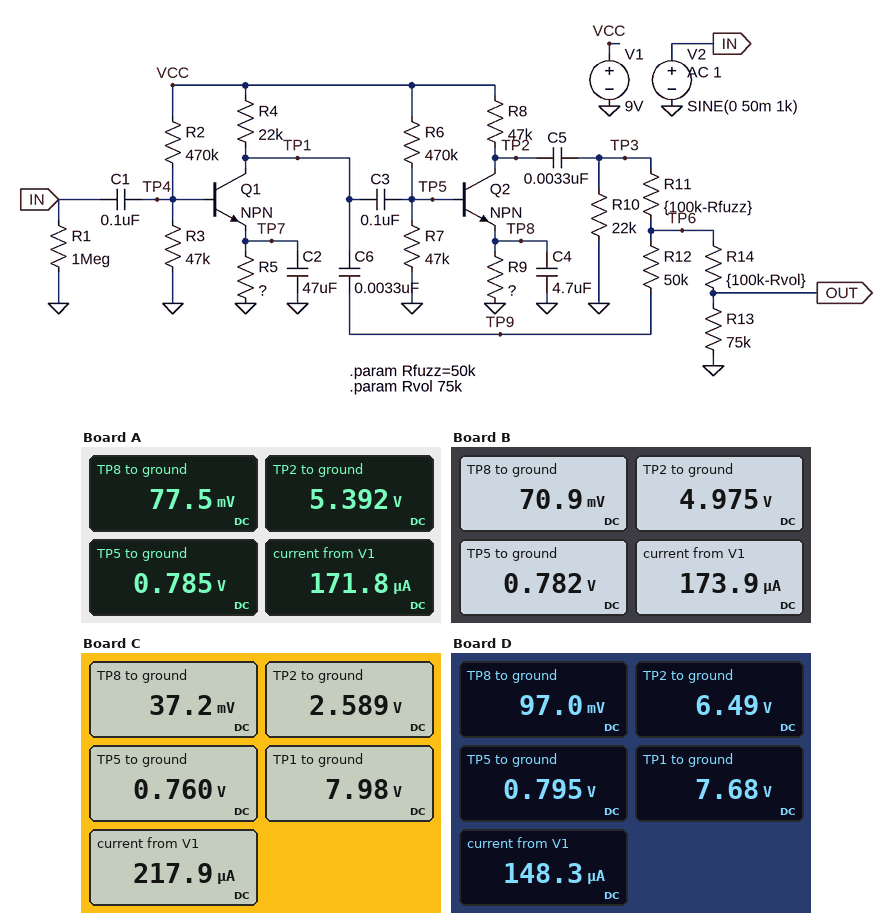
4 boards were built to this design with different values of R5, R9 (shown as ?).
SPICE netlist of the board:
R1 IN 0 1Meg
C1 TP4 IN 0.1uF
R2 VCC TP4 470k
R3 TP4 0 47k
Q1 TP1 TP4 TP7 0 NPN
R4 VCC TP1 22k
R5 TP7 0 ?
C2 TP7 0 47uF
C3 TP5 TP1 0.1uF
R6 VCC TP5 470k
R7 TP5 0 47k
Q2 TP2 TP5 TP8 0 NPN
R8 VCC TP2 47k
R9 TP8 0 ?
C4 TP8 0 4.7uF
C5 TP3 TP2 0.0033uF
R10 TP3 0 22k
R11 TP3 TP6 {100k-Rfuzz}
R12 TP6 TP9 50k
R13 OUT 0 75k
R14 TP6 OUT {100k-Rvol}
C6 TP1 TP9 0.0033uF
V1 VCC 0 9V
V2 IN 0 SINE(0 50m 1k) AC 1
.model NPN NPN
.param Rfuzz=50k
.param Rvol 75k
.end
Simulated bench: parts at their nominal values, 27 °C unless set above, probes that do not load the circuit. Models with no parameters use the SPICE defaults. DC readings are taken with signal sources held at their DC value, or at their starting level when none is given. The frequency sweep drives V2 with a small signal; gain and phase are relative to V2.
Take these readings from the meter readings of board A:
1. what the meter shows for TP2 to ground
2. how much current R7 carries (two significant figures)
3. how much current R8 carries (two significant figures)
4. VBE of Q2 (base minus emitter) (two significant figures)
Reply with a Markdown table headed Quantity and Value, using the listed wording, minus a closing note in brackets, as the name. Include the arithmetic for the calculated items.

| Quantity | Value |
|---|---|
| what the meter shows for TP2 to ground | 5.392 V |
| how much current R7 carries | (785 mV) / 47 kΩ = 17 µA |
| how much current R8 carries | (9 V - 5.392 V) / 47 kΩ = 77 µA |
| VBE of Q2 (base minus emitter) | 785 mV - 77.5 mV = 710 mV |
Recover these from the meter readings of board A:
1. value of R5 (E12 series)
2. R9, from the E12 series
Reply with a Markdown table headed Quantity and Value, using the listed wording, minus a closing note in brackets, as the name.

| Quantity | Value |
|---|---|
| value of R5 | 1.5 kΩ |
| R9, from the E12 series | 1 kΩ |
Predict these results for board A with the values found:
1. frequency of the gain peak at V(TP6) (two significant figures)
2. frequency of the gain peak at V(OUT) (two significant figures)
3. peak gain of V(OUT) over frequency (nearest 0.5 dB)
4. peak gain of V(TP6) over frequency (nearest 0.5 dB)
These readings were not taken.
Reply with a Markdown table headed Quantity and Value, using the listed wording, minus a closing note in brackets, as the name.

| Quantity | Value |
|---|---|
| frequency of the gain peak at V(TP6) | 340 Hz |
| frequency of the gain peak at V(OUT) | 340 Hz |
| peak gain of V(OUT) over frequency | 47.0 dB |
| peak gain of V(TP6) over frequency | 49.5 dB |
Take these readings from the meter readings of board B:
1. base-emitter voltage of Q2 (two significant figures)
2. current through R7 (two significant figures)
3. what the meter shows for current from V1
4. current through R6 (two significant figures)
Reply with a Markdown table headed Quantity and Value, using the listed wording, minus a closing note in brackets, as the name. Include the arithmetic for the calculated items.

| Quantity | Value |
|---|---|
| base-emitter voltage of Q2 | 782 mV - 70.9 mV = 710 mV |
| current through R7 | (782 mV) / 47 kΩ = 17 µA |
| what the meter shows for current from V1 | 173.9 µA |
| current through R6 | (9 V - 782 mV) / 470 kΩ = 17 µA |
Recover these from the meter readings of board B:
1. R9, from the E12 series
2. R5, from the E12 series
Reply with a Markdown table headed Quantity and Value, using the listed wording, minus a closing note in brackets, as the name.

| Quantity | Value |
|---|---|
| R9, from the E12 series | 820 Ω |
| R5, from the E12 series | 1.8 kΩ |
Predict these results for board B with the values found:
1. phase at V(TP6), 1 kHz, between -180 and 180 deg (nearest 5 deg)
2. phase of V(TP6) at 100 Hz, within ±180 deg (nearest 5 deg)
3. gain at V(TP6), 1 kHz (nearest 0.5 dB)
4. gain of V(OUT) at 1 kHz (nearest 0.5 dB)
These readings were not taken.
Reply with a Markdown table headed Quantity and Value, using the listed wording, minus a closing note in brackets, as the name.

| Quantity | Value |
|---|---|
| phase at V(TP6), 1 kHz, between -180 and 180 deg | -20 deg |
| phase of V(TP6) at 100 Hz, within ±180 deg | 165 deg |
| gain at V(TP6), 1 kHz | 41.0 dB |
| gain of V(OUT) at 1 kHz | 38.5 dB |
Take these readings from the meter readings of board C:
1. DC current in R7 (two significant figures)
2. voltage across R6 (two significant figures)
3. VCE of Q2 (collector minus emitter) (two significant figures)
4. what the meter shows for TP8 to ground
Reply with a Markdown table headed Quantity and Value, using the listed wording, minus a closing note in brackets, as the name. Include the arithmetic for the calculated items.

| Quantity | Value |
|---|---|
| DC current in R7 | (760 mV) / 47 kΩ = 16 µA |
| voltage across R6 | 9 V - 760 mV = 8.2 V |
| VCE of Q2 (collector minus emitter) | 2.589 V - 37.2 mV = 2.6 V |
| what the meter shows for TP8 to ground | 37.2 mV |
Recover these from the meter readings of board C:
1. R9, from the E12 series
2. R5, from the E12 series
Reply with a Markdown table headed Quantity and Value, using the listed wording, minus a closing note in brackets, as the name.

| Quantity | Value |
|---|---|
| R9, from the E12 series | 270 Ω |
| R5, from the E12 series | 2.2 kΩ |
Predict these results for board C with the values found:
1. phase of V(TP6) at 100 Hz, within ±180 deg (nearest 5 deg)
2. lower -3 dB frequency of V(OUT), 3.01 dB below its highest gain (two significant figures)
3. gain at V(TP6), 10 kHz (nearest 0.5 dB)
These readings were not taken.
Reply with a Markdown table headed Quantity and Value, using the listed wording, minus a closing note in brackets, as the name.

| Quantity | Value |
|---|---|
| phase of V(TP6) at 100 Hz, within ±180 deg | 150 deg |
| lower -3 dB frequency of V(OUT), 3.01 dB below its highest gain | 240 Hz |
| gain at V(TP6), 10 kHz | 37.0 dB |
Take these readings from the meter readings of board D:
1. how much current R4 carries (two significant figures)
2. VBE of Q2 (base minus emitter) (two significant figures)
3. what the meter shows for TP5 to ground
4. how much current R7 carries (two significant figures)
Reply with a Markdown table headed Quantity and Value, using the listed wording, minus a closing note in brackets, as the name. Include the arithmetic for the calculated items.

| Quantity | Value |
|---|---|
| how much current R4 carries | (9 V - 7.68 V) / 22 kΩ = 60 µA |
| VBE of Q2 (base minus emitter) | 795 mV - 97 mV = 700 mV |
| what the meter shows for TP5 to ground | 0.795 V |
| how much current R7 carries | (795 mV) / 47 kΩ = 17 µA |
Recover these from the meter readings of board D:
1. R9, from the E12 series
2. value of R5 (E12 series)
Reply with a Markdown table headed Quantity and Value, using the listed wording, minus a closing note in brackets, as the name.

| Quantity | Value |
|---|---|
| R9, from the E12 series | 1.8 kΩ |
| value of R5 | 1.5 kΩ |
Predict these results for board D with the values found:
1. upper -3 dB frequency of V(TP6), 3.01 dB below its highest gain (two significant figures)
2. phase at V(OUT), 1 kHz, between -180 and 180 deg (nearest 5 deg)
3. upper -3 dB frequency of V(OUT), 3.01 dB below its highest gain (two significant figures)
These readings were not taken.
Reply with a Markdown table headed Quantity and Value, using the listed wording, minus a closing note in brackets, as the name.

| Quantity | Value |
|---|---|
| upper -3 dB frequency of V(TP6), 3.01 dB below its highest gain | 640 Hz |
| phase at V(OUT), 1 kHz, between -180 and 180 deg | -15 deg |
| upper -3 dB frequency of V(OUT), 3.01 dB below its highest gain | 640 Hz |
